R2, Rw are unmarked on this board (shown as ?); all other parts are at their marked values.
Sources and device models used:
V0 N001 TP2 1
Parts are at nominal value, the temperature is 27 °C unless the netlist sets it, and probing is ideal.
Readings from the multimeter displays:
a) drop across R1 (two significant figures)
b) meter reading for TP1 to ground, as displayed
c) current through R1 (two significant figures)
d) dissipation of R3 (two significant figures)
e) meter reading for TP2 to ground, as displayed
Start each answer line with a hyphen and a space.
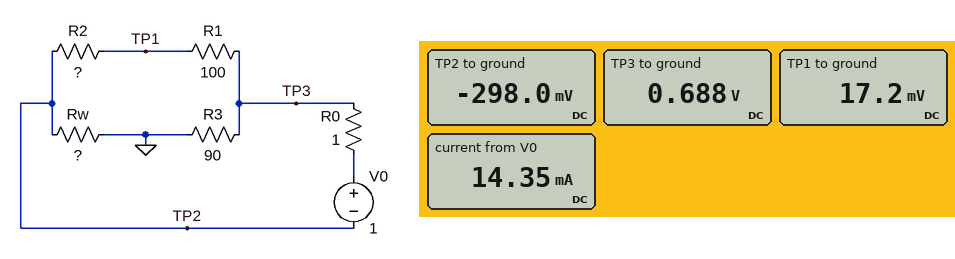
- 670 mV
- 17.2 mV
- 6.7 mA
- 5.3 mW
- -298.0 mV
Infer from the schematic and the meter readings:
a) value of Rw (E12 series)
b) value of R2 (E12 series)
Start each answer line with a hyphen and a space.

- 39 Ω
- 47 Ω
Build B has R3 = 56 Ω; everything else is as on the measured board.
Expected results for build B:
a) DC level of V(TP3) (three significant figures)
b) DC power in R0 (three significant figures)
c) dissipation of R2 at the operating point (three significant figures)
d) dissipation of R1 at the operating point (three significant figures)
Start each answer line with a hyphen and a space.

- 579 mV
- 290 µW
- 2.10 mW
- 4.47 mW
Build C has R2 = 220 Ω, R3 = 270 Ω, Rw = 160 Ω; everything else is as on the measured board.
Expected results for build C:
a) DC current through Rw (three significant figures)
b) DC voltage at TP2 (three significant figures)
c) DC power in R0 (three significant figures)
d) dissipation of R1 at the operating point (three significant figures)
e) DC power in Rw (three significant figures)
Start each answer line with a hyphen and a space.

- 2.31 mA
- -370 mV
- 29.4 µW
- 966 µW
- 856 µW
